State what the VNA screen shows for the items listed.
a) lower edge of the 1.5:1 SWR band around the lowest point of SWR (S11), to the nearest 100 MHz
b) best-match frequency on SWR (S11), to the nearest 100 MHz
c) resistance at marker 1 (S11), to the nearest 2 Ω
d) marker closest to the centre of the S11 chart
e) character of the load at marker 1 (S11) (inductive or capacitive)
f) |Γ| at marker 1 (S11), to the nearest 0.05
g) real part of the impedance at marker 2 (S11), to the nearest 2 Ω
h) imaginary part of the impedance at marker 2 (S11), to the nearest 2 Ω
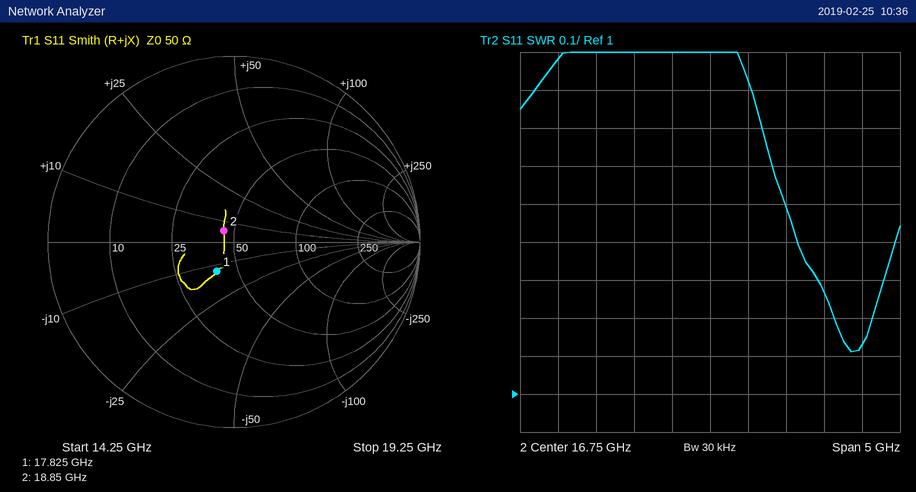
17.7 GHz
18.6 GHz
40 Ω
marker 2
capacitive
0.20
44 Ω
+6 Ω
